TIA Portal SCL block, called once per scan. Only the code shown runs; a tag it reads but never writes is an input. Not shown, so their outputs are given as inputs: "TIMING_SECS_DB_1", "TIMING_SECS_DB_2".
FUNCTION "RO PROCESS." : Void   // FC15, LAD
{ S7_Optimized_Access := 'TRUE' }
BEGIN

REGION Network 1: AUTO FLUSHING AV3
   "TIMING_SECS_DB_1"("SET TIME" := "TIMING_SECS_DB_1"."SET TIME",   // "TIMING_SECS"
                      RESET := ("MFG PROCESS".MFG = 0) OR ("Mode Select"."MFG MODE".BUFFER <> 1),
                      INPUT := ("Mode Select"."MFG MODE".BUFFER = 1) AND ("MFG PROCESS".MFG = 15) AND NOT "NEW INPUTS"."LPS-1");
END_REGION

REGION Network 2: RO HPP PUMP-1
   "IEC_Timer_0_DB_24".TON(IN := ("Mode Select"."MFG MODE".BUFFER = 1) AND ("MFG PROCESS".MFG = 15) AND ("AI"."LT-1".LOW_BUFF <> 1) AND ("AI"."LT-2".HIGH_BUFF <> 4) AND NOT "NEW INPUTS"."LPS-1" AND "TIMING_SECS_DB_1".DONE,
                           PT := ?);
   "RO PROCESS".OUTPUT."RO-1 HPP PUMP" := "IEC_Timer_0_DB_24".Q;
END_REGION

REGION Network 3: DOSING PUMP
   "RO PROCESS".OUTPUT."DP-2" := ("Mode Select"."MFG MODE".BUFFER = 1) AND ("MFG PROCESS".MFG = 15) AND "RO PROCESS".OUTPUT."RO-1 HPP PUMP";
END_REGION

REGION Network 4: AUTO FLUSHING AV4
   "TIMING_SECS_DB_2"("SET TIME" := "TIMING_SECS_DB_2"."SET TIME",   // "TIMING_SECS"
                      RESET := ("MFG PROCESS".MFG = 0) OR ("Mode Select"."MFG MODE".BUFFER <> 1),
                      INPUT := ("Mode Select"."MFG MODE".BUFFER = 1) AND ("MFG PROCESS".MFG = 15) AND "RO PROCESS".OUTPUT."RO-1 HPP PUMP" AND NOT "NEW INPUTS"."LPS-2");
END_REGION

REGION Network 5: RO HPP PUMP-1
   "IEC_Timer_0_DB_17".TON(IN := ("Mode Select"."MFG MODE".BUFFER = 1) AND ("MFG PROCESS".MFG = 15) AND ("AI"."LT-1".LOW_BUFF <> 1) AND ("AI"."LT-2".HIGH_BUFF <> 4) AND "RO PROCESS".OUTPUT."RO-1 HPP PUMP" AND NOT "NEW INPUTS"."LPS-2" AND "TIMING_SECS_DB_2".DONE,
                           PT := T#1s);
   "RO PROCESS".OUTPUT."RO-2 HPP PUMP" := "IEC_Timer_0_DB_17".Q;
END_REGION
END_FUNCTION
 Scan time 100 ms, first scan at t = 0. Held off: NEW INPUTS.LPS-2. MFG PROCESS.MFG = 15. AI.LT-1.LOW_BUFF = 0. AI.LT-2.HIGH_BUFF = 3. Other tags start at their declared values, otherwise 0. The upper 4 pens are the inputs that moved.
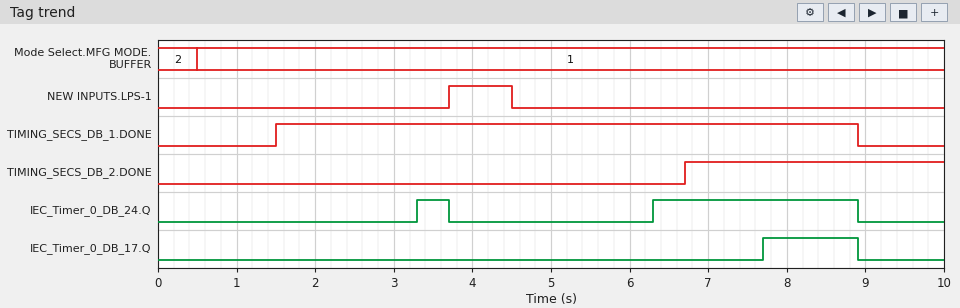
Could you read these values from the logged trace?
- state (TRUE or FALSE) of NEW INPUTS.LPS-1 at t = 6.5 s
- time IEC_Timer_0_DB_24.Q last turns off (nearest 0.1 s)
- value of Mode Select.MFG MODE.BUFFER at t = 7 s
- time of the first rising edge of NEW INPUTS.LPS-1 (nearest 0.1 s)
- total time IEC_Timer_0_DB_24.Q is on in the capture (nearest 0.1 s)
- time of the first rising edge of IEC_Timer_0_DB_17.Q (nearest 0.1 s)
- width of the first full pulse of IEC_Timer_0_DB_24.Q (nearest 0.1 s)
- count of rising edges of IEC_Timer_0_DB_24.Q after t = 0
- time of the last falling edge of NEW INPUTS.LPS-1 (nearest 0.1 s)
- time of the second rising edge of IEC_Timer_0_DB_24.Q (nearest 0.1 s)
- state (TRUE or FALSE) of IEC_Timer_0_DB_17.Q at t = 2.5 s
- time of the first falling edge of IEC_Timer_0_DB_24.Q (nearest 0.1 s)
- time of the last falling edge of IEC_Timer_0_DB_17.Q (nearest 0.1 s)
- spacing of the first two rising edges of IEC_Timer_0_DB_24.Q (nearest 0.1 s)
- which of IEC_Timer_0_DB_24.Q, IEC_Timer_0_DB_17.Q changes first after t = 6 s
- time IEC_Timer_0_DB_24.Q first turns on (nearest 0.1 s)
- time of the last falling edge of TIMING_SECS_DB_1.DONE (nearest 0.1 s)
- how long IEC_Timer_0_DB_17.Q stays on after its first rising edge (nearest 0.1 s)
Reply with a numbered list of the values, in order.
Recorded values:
1. FALSE
2. 8.9 s
3. 1
4. 3.7 s
5. 3.0 s
6. 7.7 s
7. 0.4 s
8. 2
9. 4.5 s
10. 6.3 s
11. FALSE
12. 3.7 s
13. 8.9 s
14. 3.0 s
15. IEC_Timer_0_DB_24.Q
16. 3.3 s
17. 8.9 s
18. 1.2 s
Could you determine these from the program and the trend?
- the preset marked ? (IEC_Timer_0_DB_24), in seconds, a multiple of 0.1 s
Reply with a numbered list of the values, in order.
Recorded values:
1. 1.8 s
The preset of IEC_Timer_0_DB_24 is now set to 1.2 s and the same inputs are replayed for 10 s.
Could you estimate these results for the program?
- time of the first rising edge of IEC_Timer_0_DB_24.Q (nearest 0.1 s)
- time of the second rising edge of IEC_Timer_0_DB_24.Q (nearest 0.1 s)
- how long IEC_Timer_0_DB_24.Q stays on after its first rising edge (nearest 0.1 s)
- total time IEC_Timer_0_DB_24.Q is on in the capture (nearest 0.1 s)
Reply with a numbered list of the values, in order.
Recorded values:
1. 2.7 s
2. 5.7 s
3. 1.0 s
4. 4.2 s
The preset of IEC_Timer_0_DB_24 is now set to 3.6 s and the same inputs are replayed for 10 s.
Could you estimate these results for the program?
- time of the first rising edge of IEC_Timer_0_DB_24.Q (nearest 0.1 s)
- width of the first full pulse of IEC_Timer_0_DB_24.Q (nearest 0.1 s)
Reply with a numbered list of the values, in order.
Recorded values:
1. 8.1 s
2. 0.8 s
